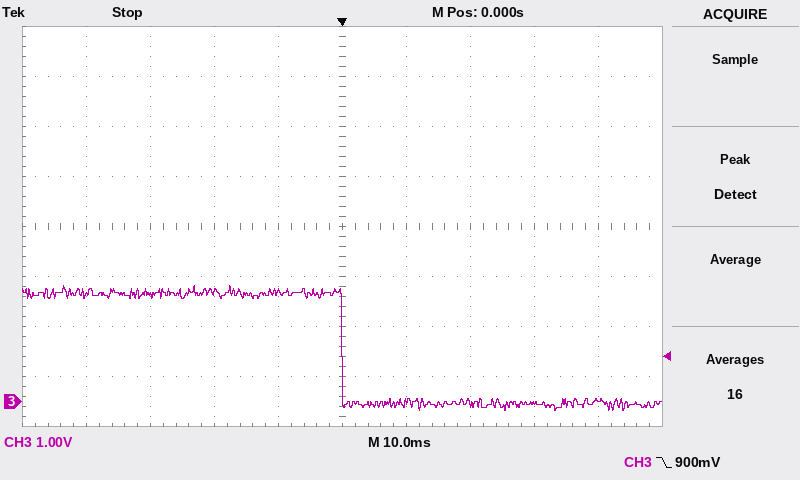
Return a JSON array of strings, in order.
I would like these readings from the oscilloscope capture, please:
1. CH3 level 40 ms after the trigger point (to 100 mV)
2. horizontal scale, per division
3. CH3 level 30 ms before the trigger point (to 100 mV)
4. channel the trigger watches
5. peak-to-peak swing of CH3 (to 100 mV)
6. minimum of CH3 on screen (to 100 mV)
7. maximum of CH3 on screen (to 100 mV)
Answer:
["0.0 V", "10 ms", "2.1 V", "CH3", "2.5 V", "-200 mV", "2.3 V"]
